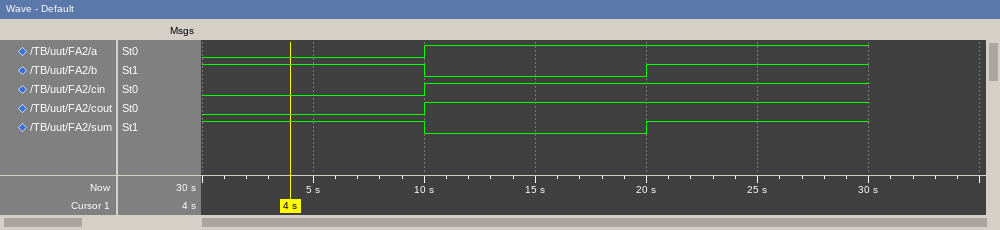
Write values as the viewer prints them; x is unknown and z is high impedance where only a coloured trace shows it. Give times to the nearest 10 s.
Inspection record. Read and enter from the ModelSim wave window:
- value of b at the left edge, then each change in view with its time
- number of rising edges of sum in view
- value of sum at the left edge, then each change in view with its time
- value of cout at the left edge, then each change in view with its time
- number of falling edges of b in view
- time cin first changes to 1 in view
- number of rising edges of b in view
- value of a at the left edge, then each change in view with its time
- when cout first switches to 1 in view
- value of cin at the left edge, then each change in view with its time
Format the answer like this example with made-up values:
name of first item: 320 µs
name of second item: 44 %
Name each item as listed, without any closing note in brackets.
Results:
value of b at the left edge, then each change in view with its time: 1, 0 at 10 s, 1 at 20 s
number of rising edges of sum in view: 1
value of sum at the left edge, then each change in view with its time: 1, 0 at 10 s, 1 at 20 s
value of cout at the left edge, then each change in view with its time: 0, 1 at 10 s
number of falling edges of b in view: 1
time cin first changes to 1 in view: 10 s
number of rising edges of b in view: 1
value of a at the left edge, then each change in view with its time: 0, 1 at 10 s
when cout first switches to 1 in view: 10 s
value of cin at the left edge, then each change in view with its time: 0, 1 at 10 s
